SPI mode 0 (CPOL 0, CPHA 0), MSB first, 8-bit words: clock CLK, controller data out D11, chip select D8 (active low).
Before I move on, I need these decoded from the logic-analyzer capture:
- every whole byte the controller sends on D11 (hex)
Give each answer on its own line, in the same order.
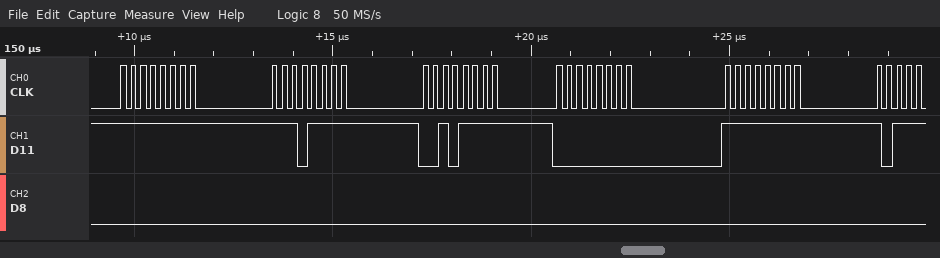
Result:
FF EF 2F 00 FF
